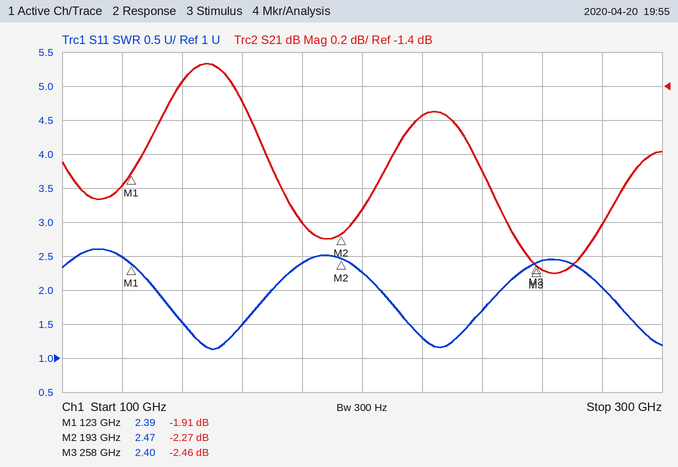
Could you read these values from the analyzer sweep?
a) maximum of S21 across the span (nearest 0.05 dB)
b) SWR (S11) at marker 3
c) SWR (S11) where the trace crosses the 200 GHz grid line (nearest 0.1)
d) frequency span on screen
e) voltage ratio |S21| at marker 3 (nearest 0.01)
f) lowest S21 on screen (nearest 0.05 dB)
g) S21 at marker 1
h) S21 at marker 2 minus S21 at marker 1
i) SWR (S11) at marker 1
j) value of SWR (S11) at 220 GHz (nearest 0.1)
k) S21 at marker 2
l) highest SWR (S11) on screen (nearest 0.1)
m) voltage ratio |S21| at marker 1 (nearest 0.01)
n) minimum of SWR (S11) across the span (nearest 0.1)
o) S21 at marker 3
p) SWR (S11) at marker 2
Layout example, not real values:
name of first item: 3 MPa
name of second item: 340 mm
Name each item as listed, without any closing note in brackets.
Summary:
maximum of S21 across the span: -1.25 dB
SWR (S11) at marker 3: 2.40
SWR (S11) where the trace crosses the 200 GHz grid line: 2.3
frequency span on screen: 200 GHz
voltage ratio |S21| at marker 3: 0.75
lowest S21 on screen: -2.50 dB
S21 at marker 1: -1.91 dB
S21 at marker 2 minus S21 at marker 1: -0.36 dB
SWR (S11) at marker 1: 2.39
value of SWR (S11) at 220 GHz: 1.3
S21 at marker 2: -2.27 dB
highest SWR (S11) on screen: 2.6
voltage ratio |S21| at marker 1: 0.80
minimum of SWR (S11) across the span: 1.1
S21 at marker 3: -2.46 dB
SWR (S11) at marker 2: 2.47
